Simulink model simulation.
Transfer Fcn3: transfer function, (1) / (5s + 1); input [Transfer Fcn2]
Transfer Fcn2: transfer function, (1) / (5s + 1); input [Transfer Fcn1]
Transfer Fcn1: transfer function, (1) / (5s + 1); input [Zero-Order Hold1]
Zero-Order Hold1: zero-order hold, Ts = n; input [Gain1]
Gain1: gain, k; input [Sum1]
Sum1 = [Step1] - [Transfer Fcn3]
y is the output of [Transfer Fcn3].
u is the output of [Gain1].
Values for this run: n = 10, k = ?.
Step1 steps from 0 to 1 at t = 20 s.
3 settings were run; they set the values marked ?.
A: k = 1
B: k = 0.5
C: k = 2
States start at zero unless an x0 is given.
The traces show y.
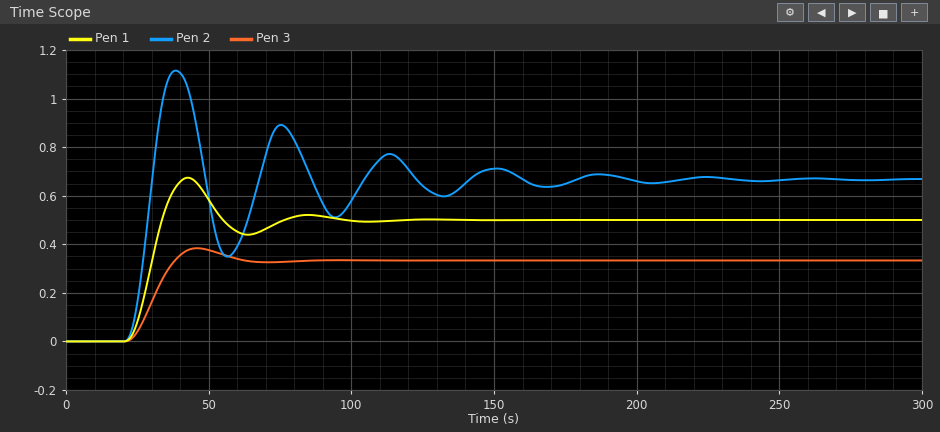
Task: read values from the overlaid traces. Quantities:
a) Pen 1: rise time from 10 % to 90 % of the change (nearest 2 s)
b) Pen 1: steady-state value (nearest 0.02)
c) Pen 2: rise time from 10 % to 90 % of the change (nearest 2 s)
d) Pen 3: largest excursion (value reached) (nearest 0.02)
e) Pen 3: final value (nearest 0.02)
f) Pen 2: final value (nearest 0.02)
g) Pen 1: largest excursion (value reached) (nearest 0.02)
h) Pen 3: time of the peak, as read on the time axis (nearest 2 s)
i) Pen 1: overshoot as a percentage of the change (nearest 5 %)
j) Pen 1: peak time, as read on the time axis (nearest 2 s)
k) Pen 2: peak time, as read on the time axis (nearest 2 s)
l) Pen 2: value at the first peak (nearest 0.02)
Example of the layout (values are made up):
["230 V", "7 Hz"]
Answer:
["8 s", "0.50", "6 s", "0.38", "0.34", "0.66", "0.68", "46 s", "35 %", "42 s", "38 s", "1.12"]
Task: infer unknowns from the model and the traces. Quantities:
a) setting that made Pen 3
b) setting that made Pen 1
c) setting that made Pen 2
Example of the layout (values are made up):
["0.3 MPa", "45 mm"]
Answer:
["B", "A", "C"]
